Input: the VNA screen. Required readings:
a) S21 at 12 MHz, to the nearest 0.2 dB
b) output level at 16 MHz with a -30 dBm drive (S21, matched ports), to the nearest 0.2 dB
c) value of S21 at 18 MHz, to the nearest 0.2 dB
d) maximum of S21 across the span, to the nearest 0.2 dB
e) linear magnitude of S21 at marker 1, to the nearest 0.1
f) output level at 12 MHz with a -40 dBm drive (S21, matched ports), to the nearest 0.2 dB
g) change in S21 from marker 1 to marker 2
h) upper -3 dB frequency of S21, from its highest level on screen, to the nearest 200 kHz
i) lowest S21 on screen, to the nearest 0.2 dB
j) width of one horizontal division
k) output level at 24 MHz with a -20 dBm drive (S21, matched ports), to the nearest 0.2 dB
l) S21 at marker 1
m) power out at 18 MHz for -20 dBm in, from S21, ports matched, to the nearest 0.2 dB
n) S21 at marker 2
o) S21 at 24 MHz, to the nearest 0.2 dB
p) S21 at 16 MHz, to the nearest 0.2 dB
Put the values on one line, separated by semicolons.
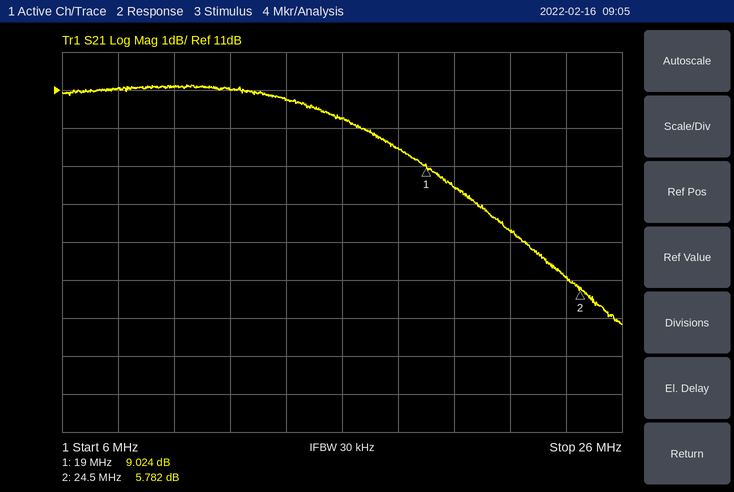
11.0 dB; -19.8 dBm; 9.4 dB; 11.2 dB; 2.8; -29.0 dBm; -3.242 dB; 20.6 MHz; 4.8 dB; 2 MHz; -14.0 dBm; 9.024 dB; -10.6 dBm; 5.782 dB; 6.0 dB; 10.2 dB
